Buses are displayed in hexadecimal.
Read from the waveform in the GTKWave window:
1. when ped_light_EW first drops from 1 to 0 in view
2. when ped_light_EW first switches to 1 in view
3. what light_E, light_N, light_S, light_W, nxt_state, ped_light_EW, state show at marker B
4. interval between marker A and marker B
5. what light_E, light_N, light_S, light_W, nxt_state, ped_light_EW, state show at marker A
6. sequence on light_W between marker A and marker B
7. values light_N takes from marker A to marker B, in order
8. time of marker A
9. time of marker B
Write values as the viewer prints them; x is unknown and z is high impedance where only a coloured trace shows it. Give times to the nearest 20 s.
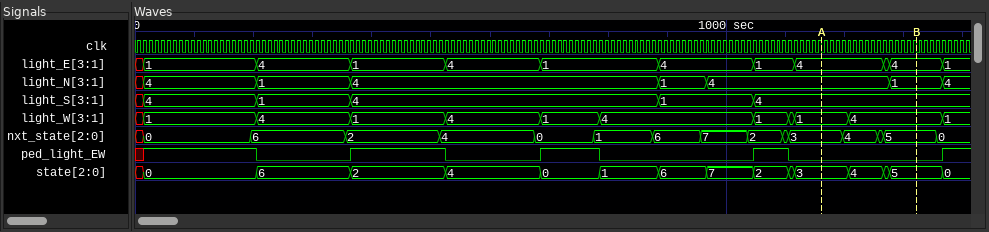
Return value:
200 s
20 s
light_E=4, light_N=1, light_S=4, light_W=4, nxt_state=5, ped_light_EW=0, state=5
160 s
light_E=4, light_N=4, light_S=4, light_W=1, nxt_state=3, ped_light_EW=0, state=3
1, 4
4, 1
1160 s
1320 s
